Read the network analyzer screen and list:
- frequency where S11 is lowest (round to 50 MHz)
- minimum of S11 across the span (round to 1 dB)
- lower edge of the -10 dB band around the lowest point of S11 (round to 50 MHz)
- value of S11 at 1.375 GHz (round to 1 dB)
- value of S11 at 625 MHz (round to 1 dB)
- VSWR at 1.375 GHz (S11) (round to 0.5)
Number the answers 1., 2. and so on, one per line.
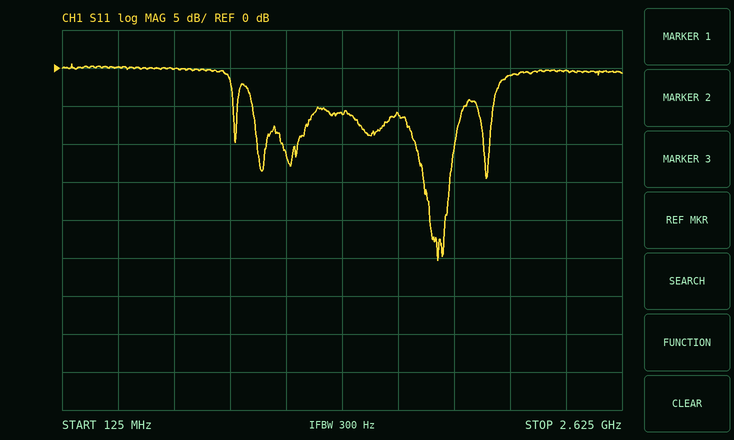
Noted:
1. 1.80 GHz
2. -25 dB
3. 1.70 GHz
4. -6 dB
5. 0 dB
6. 3.0
